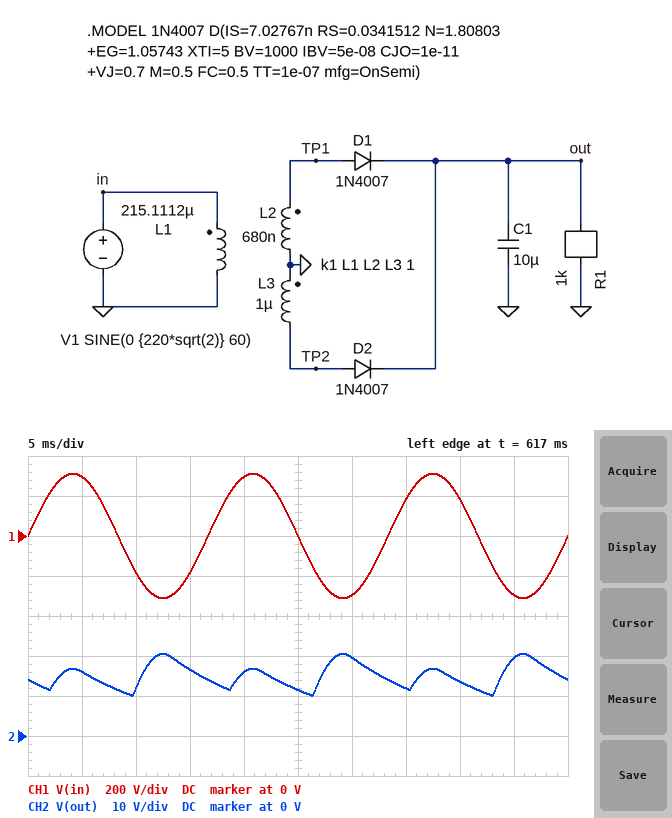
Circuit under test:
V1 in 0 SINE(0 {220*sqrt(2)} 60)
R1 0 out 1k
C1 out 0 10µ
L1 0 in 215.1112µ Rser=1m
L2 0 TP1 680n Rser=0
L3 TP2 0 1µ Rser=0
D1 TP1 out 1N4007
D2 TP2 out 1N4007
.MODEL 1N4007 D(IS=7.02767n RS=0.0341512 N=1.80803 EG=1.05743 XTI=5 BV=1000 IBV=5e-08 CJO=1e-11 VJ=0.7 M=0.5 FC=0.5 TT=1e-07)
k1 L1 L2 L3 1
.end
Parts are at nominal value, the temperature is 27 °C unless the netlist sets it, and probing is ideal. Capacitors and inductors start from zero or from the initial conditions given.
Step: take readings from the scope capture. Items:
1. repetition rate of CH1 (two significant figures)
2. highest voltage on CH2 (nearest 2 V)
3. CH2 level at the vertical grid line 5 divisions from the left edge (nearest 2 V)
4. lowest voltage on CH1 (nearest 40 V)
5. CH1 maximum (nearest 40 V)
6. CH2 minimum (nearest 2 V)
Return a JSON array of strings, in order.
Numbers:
["60 Hz", "20 V", "12 V", "-320 V", "320 V", "10 V"]
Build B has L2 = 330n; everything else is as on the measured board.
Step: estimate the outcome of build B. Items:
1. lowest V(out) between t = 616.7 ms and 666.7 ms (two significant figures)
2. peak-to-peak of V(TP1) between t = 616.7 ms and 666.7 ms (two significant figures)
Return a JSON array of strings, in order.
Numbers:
["7.2 V", "24 V"]
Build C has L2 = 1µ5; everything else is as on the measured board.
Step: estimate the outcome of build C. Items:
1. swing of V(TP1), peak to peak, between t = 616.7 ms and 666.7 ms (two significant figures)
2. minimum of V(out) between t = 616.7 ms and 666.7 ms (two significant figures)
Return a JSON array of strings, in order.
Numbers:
["52 V", "12 V"]
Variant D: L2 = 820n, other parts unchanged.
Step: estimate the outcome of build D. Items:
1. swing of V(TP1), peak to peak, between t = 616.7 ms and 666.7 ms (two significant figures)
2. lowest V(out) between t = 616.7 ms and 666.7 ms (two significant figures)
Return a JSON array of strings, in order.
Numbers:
["38 V", "11 V"]
